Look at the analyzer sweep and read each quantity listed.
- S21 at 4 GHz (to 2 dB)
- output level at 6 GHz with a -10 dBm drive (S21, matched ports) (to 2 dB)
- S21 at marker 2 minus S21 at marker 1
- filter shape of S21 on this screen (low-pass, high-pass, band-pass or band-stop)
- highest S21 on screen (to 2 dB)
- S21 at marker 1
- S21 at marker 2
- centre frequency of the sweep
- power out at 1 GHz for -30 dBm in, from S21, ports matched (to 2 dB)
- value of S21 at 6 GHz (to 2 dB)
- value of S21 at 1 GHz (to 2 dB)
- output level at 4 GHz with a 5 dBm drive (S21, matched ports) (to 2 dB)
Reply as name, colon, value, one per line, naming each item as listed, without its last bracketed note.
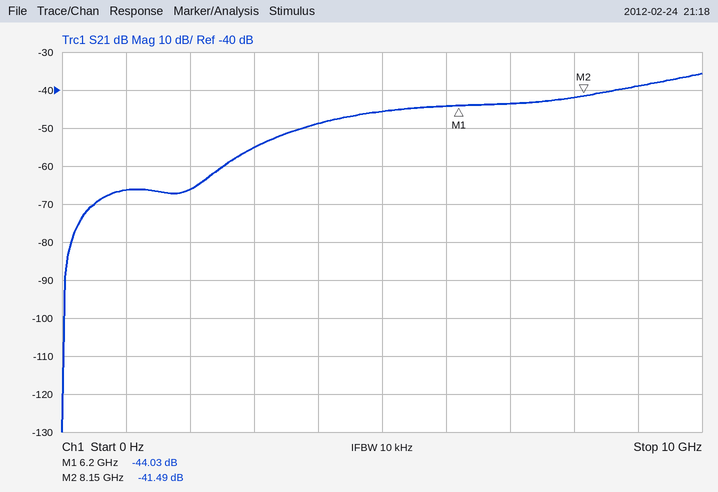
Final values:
S21 at 4 GHz: -48 dB
output level at 6 GHz with a -10 dBm drive (S21, matched ports): -54 dBm
S21 at marker 2 minus S21 at marker 1: 2.54 dB
filter shape of S21 on this screen: high-pass
highest S21 on screen: -36 dB
S21 at marker 1: -44.03 dB
S21 at marker 2: -41.49 dB
centre frequency of the sweep: 5 GHz
power out at 1 GHz for -30 dBm in, from S21, ports matched: -96 dBm
value of S21 at 6 GHz: -44 dB
value of S21 at 1 GHz: -66 dB
output level at 4 GHz with a 5 dBm drive (S21, matched ports): -44 dBm
